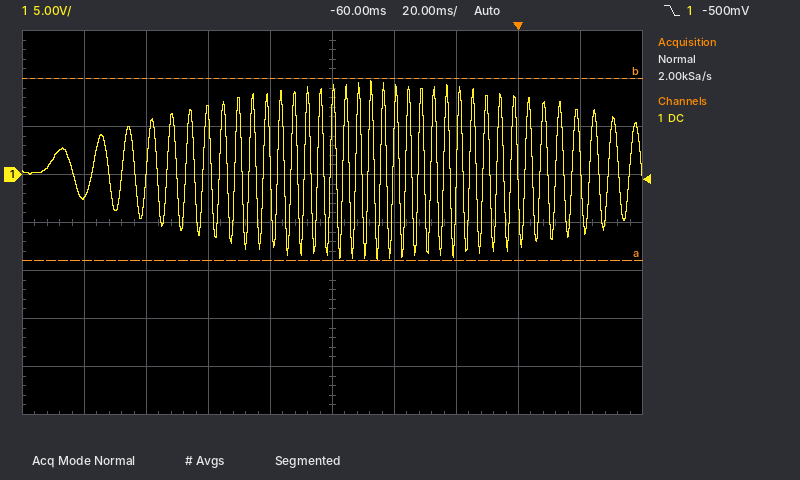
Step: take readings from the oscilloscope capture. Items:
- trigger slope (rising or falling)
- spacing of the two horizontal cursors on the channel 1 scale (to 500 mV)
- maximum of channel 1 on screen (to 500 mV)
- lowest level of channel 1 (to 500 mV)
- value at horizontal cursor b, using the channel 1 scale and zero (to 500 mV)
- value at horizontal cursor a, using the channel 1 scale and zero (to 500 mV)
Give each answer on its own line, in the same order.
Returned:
falling
19.0 V
10.0 V
-9.0 V
10.0 V
-9.0 V
